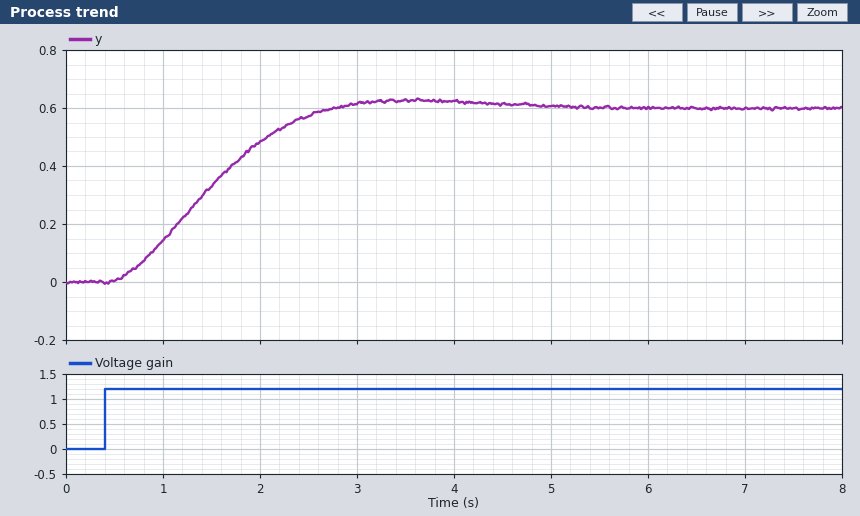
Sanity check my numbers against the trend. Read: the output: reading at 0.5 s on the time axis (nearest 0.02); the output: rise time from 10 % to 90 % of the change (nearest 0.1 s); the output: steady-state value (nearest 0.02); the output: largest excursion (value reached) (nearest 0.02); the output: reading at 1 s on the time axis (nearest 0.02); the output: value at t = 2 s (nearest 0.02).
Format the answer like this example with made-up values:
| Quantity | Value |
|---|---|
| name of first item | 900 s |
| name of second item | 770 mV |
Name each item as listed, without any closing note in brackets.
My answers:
| Quantity | Value |
|---|---|
| the output: reading at 0.5 s on the time axis | 0.00 |
| the output: rise time from 10 % to 90 % of the change | 1.5 s |
| the output: steady-state value | 0.60 |
| the output: largest excursion (value reached) | 0.62 |
| the output: reading at 1 s on the time axis | 0.14 |
| the output: value at t = 2 s | 0.48 |
